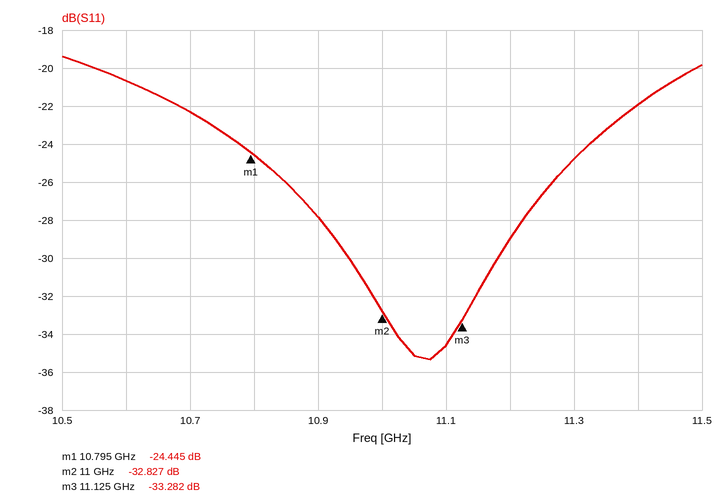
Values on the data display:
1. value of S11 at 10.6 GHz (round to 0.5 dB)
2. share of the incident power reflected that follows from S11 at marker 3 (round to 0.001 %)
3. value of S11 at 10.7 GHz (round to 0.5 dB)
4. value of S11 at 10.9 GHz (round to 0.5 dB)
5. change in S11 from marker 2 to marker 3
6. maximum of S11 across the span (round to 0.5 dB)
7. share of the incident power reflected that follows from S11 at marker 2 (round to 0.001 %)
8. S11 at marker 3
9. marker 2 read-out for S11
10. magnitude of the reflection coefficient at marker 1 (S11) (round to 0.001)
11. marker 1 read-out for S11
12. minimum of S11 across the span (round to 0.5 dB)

-20.5 dB
0.047 %
-22.5 dB
-28.0 dB
-0.455 dB
-19.5 dB
0.052 %
-33.282 dB
-32.827 dB
0.060
-24.445 dB
-35.5 dB
